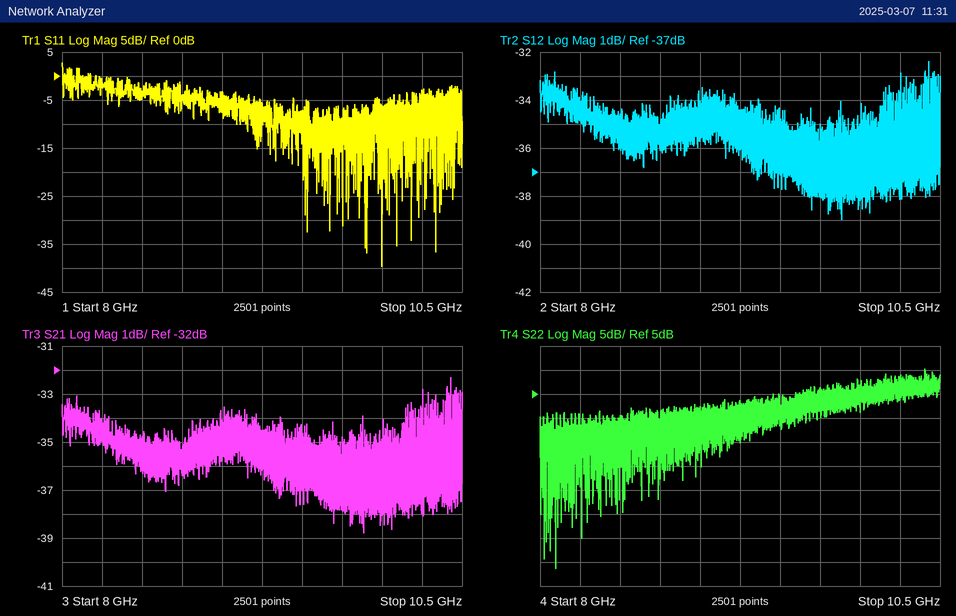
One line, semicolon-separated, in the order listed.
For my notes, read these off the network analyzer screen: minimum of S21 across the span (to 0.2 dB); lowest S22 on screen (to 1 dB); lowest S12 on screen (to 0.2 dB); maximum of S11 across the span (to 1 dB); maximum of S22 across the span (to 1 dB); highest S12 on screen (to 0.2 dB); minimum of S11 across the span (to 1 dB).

-38.8 dB; -31 dB; -39.0 dB; 3 dB; 10 dB; -32.4 dB; -40 dB
